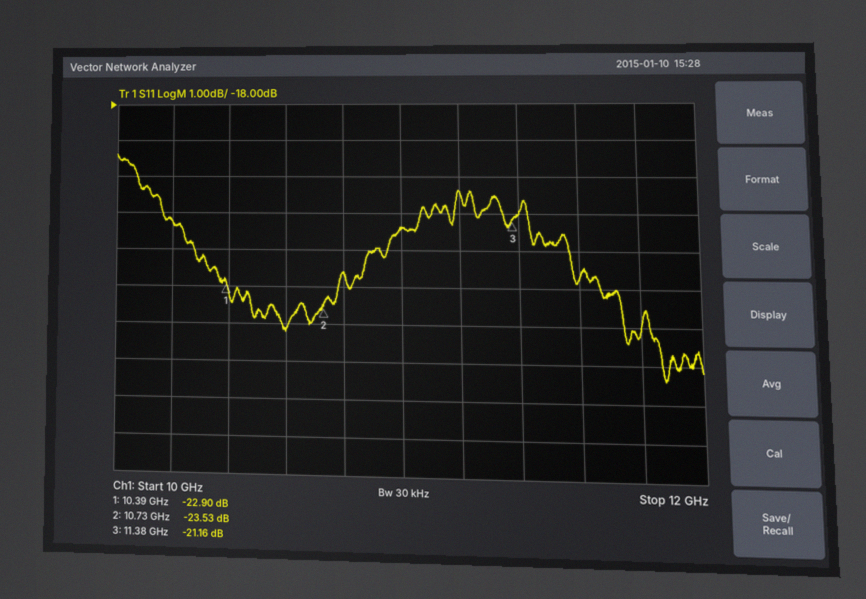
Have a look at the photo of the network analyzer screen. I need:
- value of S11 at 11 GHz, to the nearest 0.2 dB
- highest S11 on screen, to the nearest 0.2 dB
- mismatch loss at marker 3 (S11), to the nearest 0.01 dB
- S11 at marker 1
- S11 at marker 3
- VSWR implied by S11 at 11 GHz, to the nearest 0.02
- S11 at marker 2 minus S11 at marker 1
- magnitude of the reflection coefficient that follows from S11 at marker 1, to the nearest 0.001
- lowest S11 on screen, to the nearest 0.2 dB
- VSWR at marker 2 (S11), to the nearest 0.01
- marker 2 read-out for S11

-21.4 dB
-19.4 dB
0.03 dB
-22.90 dB
-21.16 dB
1.18
-0.63 dB
0.072
-25.4 dB
1.14
-23.53 dB
